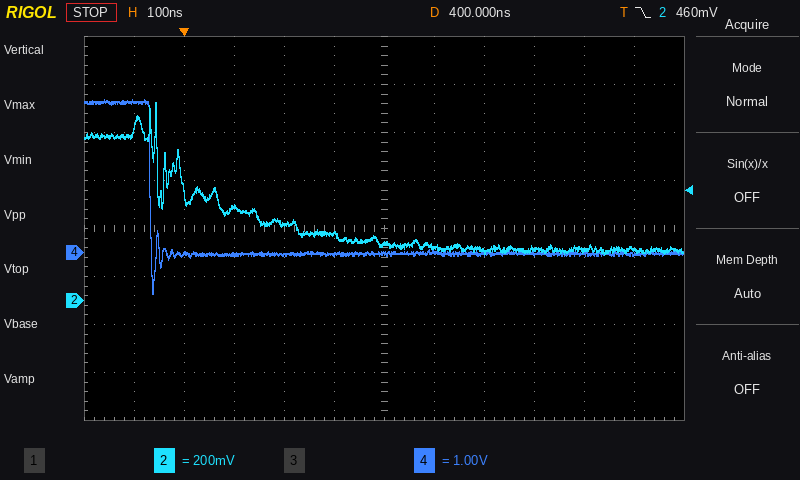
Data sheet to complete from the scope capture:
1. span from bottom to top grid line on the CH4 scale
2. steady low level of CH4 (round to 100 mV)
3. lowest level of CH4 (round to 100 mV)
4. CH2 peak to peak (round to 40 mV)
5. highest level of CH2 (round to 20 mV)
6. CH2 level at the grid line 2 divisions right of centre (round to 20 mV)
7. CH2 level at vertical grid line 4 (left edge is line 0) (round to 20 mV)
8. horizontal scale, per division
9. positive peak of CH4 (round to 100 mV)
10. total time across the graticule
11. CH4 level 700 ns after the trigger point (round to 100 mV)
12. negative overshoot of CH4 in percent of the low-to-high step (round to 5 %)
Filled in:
8 V
0.0 V
-900 mV
640 mV
820 mV
200 mV
320 mV
100 ns
3.2 V
1.2 µs
0.0 V
25 %
